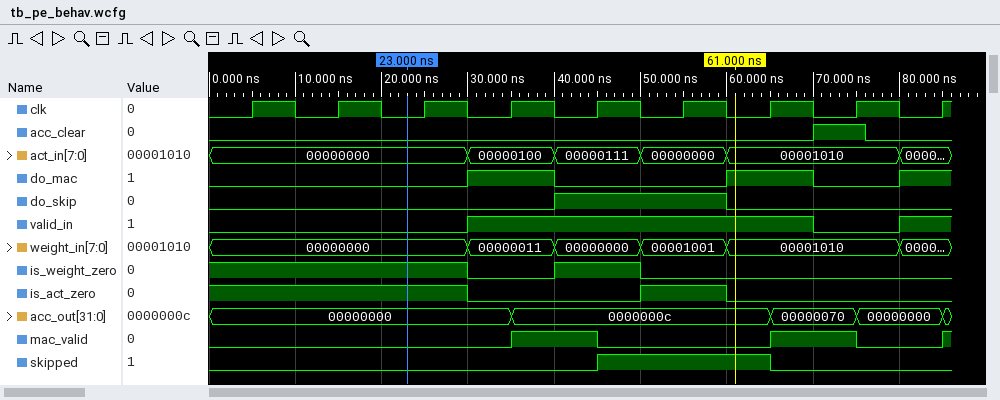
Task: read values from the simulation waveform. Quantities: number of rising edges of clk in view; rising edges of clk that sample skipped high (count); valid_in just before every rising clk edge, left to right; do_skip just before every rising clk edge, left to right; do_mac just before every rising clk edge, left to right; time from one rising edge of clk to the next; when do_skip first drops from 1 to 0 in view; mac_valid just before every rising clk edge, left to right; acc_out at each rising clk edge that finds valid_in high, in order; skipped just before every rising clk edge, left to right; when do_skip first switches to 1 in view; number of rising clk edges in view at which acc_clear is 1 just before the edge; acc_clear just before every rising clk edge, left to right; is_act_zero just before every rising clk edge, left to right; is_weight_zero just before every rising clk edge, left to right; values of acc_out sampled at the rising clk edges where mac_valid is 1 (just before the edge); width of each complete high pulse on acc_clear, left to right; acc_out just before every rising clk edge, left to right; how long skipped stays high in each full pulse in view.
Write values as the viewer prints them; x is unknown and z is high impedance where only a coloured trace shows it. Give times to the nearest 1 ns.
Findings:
9
2
0 0 0 1 1 1 1 0 1
0 0 0 0 1 1 0 0 0
0 0 0 1 0 0 1 0 1
10 ns
60 ns
0 0 0 0 1 0 0 1 0
00000000, 0000000c, 0000000c, 0000000c, 00000000
0 0 0 0 0 1 1 0 0
40 ns
1
0 0 0 0 0 0 0 1 0
1 1 1 0 0 1 0 0 0
1 1 1 0 1 0 0 0 0
0000000c, 00000070
6 ns
00000000, 00000000, 00000000, 00000000, 0000000c, 0000000c, 0000000c, 00000070, 00000000
20 ns
